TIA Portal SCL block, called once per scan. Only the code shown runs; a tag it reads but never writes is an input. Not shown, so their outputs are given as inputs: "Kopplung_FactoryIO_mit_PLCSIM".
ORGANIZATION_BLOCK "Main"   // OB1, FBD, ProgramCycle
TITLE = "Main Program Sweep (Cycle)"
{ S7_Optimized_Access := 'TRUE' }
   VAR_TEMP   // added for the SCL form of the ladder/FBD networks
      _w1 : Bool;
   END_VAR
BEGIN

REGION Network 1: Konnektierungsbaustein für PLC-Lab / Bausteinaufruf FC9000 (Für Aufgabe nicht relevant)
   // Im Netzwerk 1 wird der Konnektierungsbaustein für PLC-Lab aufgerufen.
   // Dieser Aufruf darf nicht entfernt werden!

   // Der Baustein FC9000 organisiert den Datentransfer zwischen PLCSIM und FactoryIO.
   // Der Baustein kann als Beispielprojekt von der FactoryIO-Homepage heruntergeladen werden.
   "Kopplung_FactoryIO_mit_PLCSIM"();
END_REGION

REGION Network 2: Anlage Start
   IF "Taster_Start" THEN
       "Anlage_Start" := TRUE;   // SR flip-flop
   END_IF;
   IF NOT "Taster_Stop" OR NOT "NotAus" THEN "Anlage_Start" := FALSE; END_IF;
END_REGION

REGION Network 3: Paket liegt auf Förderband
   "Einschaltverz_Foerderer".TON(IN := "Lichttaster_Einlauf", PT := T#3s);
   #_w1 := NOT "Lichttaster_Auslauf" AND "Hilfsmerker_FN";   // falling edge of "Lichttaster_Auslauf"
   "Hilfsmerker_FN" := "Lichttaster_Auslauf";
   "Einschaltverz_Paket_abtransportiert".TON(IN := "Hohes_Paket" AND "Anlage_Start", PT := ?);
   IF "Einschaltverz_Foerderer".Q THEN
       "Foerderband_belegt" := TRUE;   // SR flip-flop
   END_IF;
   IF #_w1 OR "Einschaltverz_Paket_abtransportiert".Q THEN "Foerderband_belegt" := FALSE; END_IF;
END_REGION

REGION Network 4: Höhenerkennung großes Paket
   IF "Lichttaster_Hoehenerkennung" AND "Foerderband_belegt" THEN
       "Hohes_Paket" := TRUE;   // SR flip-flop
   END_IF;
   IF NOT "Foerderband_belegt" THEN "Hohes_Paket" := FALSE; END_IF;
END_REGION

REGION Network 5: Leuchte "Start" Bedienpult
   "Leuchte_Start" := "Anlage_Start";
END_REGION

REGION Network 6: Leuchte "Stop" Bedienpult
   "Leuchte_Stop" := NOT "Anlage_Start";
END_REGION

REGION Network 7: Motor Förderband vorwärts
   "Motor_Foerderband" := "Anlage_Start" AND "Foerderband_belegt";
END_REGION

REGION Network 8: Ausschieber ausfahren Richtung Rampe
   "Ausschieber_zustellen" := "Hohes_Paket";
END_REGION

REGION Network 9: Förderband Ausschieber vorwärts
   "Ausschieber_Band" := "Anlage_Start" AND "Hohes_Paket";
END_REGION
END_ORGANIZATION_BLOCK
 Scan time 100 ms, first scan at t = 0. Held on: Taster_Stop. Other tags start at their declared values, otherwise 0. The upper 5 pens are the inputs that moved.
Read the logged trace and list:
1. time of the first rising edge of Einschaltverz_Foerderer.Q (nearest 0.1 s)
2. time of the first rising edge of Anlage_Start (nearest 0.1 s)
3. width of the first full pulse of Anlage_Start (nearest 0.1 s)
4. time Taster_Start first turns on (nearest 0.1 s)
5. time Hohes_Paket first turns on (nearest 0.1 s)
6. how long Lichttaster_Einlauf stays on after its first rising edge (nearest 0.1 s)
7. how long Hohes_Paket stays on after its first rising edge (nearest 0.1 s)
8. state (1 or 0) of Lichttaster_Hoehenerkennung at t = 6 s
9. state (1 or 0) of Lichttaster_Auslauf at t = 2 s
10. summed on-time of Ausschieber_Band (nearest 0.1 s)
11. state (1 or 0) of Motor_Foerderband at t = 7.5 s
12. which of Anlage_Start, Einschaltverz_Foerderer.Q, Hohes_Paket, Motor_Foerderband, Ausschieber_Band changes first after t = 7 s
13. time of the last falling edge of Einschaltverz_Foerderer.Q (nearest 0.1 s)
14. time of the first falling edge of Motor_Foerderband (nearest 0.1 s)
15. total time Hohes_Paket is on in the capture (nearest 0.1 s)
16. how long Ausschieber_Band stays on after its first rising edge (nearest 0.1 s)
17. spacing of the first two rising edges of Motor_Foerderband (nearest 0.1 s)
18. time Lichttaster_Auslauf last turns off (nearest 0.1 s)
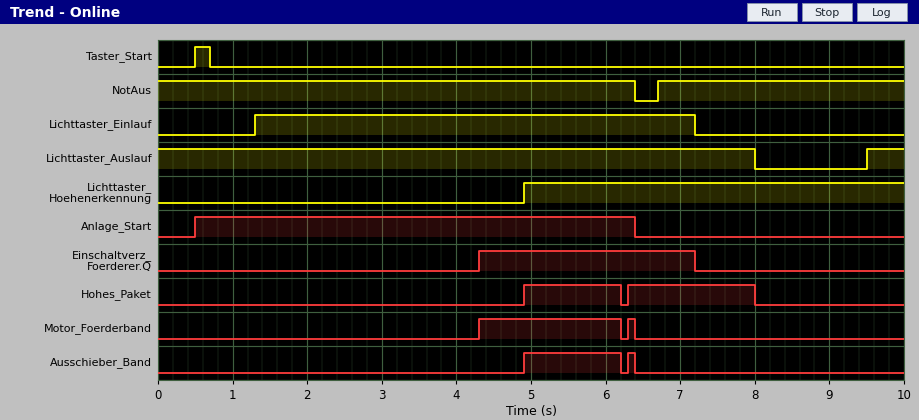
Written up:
4.3 s
0.5 s
5.9 s
0.5 s
4.9 s
5.9 s
1.3 s
1
1
1.4 s
0
Einschaltverz_Foerderer.Q
7.2 s
6.2 s
3.0 s
1.3 s
2.0 s
8.0 s
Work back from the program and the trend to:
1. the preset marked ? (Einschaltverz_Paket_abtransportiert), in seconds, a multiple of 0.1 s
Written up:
1.2 s
